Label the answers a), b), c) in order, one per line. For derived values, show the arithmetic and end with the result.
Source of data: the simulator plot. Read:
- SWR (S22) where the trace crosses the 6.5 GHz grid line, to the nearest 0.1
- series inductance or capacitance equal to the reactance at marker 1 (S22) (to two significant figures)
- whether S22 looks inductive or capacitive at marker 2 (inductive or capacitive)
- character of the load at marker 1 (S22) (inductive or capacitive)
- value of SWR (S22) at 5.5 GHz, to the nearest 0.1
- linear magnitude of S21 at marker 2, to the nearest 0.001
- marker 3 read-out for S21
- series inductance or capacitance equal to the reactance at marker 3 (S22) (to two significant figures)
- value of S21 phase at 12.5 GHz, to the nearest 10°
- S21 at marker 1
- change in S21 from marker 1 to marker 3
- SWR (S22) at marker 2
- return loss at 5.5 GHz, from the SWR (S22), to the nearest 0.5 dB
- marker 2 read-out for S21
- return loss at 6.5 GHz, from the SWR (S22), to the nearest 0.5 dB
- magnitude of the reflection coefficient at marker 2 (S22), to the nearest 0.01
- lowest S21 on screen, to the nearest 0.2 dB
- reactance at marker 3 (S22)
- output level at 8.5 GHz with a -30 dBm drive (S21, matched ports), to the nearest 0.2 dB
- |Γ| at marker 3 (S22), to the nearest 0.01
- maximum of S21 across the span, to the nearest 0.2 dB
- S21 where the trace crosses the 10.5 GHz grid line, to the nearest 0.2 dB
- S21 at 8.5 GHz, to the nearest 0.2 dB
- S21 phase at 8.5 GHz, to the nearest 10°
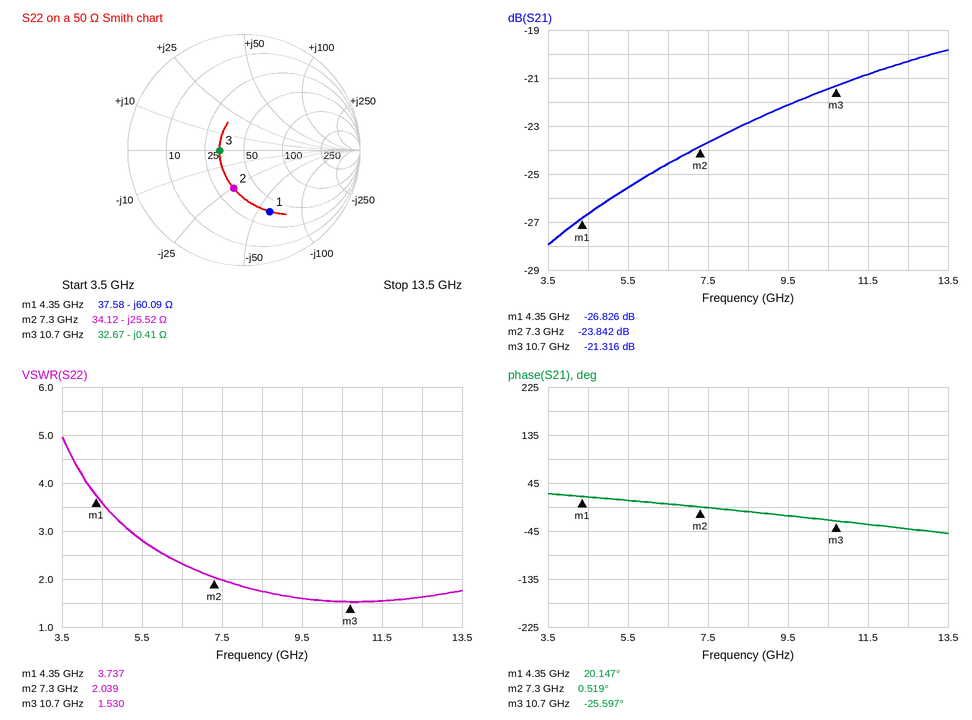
a) 2.3
b) C = 1/(2π × 4.35 GHz × 60.09 Ω) ≈ 609 fF, so 610 fF to two significant figures
c) capacitive
d) capacitive
e) 2.8
f) 10^(-23.842/20) ≈ 0.064
g) -21.316 dB
h) C = 1/(2π × 10.7 GHz × 0.41 Ω) ≈ 36 pF
i) -40°
j) -26.826 dB
k) -21.316 − (-26.826) = 5.510 dB
l) 2.039
m) −20 log10((2.8 − 1)/(2.8 + 1)) ≈ 6.5 dB
n) -23.842 dB
o) −20 log10((2.3 − 1)/(2.3 + 1)) ≈ 8.09 dB, so 8.0 dB to the nearest 0.5 dB
p) 0.34
q) -28.0 dB
r) -0.41 Ω
s) -30 dBm + (-22.8 dB) = -52.8 dBm
t) 0.21
u) -19.8 dB
v) -21.4 dB
w) -22.8 dB
x) -10°
